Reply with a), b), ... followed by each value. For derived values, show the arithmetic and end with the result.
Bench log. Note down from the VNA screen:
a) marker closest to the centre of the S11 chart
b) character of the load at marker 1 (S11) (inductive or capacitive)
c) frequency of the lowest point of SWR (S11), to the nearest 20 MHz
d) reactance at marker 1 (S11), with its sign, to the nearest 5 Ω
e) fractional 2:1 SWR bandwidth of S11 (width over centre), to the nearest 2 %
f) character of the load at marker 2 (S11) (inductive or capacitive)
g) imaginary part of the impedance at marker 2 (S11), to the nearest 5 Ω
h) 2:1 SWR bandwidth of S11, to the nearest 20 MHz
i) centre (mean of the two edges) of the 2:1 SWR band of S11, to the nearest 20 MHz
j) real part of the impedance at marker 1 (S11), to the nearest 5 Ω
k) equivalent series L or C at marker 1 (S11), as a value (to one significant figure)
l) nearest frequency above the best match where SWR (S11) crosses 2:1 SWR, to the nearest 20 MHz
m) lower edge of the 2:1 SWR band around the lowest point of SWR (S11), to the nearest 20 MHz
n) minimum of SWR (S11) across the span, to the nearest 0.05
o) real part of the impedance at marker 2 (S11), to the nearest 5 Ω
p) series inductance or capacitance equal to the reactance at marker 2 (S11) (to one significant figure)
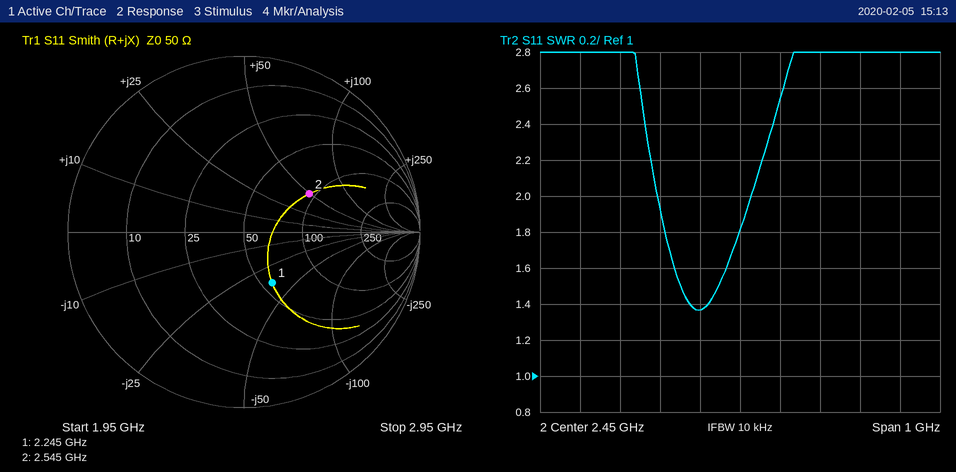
a) marker 1
b) capacitive
c) 2.34 GHz
d) -35 Ω
e) 240 MHz / 2.36 GHz ≈ 10 %
f) inductive
g) +50 Ω
h) 2.48 GHz − 2.24 GHz = 240 MHz
i) 2.36 GHz
j) 55 Ω
k) C = 1/(2π × 2.245 GHz × 35 Ω) ≈ 2 pF
l) 2.48 GHz
m) 2.24 GHz
n) 1.35
o) 90 Ω
p) L = 50 Ω/(2π × 2.545 GHz) ≈ 3 nH
